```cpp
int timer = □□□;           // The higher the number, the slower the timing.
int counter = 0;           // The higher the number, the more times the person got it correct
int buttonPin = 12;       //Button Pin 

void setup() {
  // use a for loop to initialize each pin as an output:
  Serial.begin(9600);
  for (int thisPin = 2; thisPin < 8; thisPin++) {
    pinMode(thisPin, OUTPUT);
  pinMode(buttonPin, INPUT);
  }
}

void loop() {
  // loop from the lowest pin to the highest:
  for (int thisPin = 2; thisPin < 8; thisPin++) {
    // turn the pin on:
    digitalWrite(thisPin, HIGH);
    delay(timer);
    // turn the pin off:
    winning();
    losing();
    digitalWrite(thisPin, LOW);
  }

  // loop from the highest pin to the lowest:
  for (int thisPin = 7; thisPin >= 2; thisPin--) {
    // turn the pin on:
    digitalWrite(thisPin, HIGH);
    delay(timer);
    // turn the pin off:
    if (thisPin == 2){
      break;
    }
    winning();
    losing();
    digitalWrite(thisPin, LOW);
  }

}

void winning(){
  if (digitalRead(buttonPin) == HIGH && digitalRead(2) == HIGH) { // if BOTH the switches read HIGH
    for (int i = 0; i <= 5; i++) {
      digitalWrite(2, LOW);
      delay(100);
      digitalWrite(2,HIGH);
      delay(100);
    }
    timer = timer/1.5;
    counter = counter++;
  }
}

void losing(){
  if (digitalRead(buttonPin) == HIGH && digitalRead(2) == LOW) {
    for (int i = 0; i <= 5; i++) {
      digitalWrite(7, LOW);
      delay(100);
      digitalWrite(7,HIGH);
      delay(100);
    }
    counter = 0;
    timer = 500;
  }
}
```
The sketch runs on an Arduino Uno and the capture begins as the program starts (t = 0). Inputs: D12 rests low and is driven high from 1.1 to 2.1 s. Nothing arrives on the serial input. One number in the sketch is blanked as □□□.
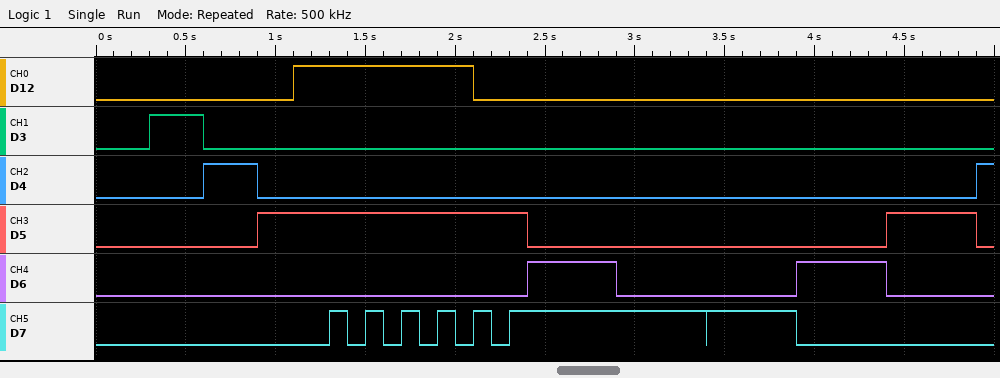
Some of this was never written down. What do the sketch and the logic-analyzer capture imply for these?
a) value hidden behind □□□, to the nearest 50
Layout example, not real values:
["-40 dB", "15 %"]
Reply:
["300"]
